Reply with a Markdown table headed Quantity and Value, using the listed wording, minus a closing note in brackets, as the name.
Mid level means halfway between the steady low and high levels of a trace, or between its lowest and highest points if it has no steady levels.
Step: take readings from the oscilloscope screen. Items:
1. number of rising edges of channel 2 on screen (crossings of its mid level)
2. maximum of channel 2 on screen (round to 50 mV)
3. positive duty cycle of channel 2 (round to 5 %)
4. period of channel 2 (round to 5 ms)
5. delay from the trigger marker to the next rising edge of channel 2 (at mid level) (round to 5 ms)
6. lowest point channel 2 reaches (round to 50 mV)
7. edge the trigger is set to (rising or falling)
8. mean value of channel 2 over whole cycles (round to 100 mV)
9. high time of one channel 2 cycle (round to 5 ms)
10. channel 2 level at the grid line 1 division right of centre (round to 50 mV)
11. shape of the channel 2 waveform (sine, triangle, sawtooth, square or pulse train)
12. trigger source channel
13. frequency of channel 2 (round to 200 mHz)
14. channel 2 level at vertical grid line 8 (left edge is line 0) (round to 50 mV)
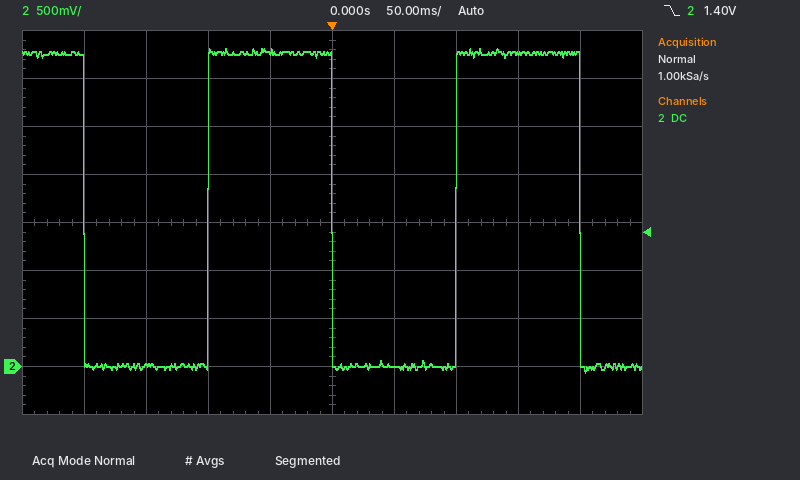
| Quantity | Value |
|---|---|
| number of rising edges of channel 2 on screen | 2 |
| maximum of channel 2 on screen | 3.30 V |
| positive duty cycle of channel 2 | 50 % |
| period of channel 2 | 200 ms |
| delay from the trigger marker to the next rising edge of channel 2 (at mid level) | 100 ms |
| lowest point channel 2 reaches | -50 mV |
| edge the trigger is set to | falling |
| mean value of channel 2 over whole cycles | 1.6 V |
| high time of one channel 2 cycle | 100 ms |
| channel 2 level at the grid line 1 division right of centre | 0 mV |
| shape of the channel 2 waveform | square |
| trigger source channel | channel 2 |
| frequency of channel 2 | 5.0 Hz |
| channel 2 level at vertical grid line 8 (left edge is line 0) | 3.25 V |
